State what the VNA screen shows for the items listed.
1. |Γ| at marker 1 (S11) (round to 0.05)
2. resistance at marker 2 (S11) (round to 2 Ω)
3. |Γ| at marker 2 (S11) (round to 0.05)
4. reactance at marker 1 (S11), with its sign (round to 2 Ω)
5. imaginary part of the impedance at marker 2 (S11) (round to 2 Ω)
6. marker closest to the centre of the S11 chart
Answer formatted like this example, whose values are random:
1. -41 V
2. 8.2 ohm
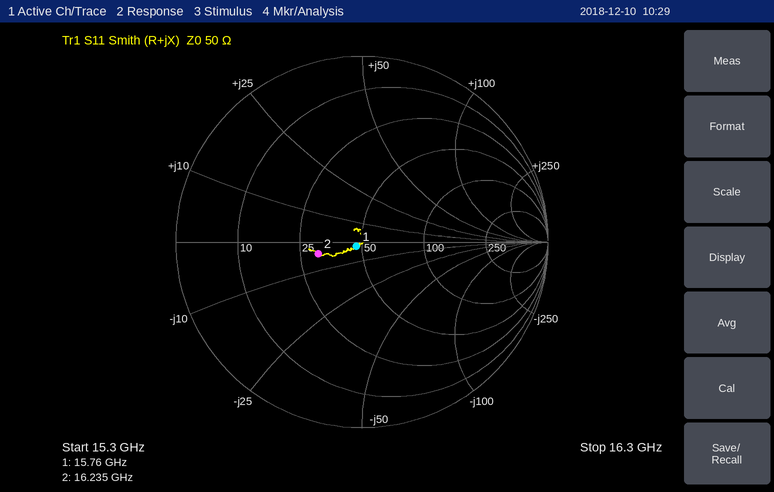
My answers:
1. 0.05
2. 30 Ω
3. 0.25
4. -2 Ω
5. -4 Ω
6. marker 1
